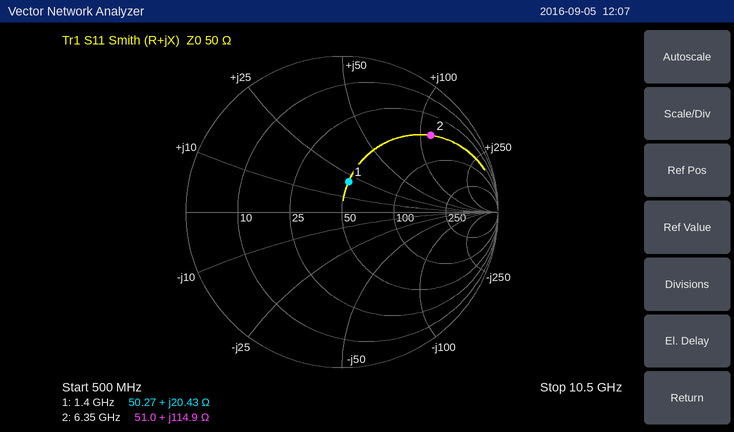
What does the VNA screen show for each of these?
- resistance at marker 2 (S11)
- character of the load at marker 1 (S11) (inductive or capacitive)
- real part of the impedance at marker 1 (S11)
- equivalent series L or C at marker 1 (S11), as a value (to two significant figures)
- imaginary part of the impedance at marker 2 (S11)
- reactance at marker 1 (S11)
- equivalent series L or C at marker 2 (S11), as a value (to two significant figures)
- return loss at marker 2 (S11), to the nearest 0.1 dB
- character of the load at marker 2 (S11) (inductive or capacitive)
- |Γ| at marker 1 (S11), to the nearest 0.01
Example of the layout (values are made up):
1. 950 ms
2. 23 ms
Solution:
1. 51.0 Ω
2. inductive
3. 50.27 Ω
4. 2.3 nH
5. +114.9 Ω
6. +20.43 Ω
7. 2.9 nH
8. 2.5 dB
9. inductive
10. 0.20
